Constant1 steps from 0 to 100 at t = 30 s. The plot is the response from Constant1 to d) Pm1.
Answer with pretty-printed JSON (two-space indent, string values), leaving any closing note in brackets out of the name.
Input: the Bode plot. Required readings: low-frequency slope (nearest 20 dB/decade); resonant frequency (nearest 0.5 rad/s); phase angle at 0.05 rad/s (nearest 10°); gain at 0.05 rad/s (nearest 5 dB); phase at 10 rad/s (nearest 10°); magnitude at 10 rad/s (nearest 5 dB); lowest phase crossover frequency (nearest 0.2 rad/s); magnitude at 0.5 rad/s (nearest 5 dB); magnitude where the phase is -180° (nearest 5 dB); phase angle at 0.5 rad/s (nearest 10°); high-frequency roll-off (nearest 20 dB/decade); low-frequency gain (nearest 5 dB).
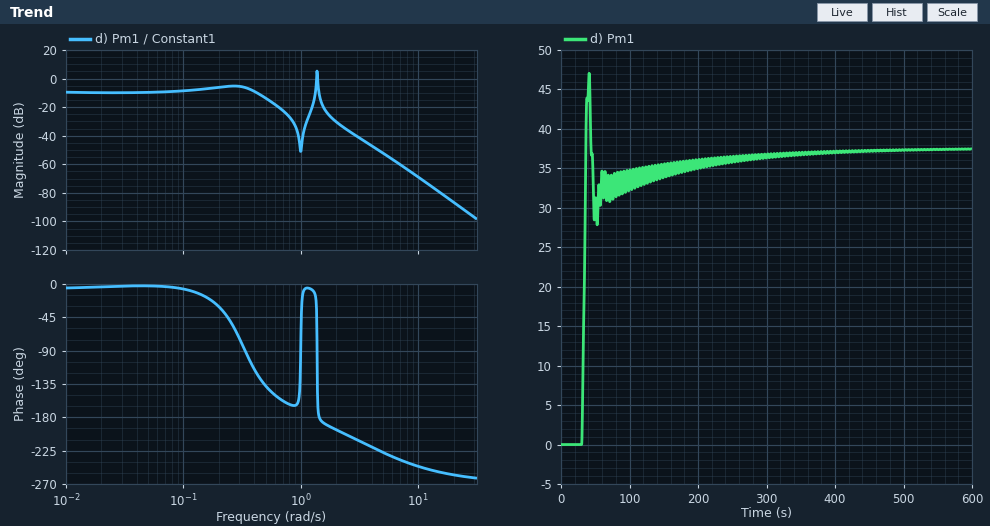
{
  "low-frequency slope": "0 dB/decade",
  "resonant frequency": "1.5 rad/s",
  "phase angle at 0.05 rad/s": "0°",
  "gain at 0.05 rad/s": "-10 dB",
  "phase at 10 rad/s": "-250°",
  "magnitude at 10 rad/s": "-70 dB",
  "lowest phase crossover frequency": "1.4 rad/s",
  "magnitude at 0.5 rad/s": "-15 dB",
  "magnitude where the phase is -180°": "-10 dB",
  "phase angle at 0.5 rad/s": "-140°",
  "high-frequency roll-off": "-60 dB/decade",
  "low-frequency gain": "-10 dB"
}
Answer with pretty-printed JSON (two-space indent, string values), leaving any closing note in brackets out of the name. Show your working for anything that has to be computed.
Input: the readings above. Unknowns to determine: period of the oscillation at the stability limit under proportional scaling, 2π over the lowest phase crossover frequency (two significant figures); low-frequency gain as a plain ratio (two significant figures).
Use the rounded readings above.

{
  "period of the oscillation at the stability limit under proportional scaling, 2π over the lowest phase crossover frequency": "2π / 1.4 = 4.5 s",
  "low-frequency gain as a plain ratio": "10^(-10 / 20) = 0.32"
}
